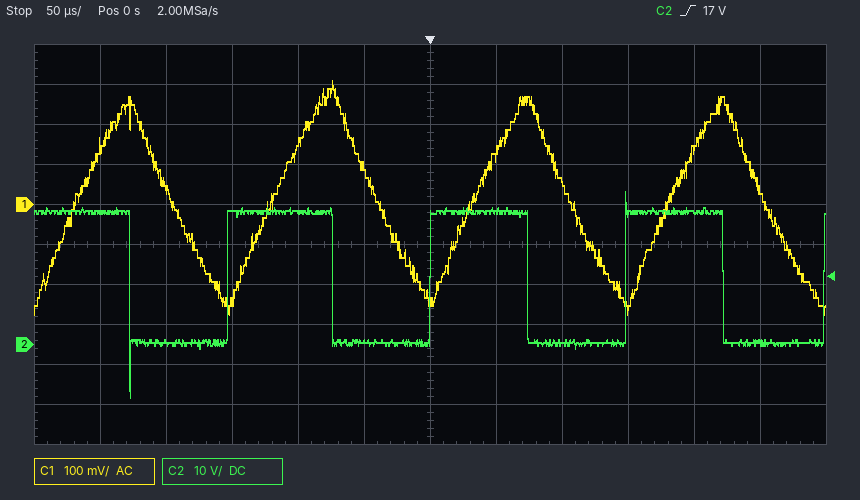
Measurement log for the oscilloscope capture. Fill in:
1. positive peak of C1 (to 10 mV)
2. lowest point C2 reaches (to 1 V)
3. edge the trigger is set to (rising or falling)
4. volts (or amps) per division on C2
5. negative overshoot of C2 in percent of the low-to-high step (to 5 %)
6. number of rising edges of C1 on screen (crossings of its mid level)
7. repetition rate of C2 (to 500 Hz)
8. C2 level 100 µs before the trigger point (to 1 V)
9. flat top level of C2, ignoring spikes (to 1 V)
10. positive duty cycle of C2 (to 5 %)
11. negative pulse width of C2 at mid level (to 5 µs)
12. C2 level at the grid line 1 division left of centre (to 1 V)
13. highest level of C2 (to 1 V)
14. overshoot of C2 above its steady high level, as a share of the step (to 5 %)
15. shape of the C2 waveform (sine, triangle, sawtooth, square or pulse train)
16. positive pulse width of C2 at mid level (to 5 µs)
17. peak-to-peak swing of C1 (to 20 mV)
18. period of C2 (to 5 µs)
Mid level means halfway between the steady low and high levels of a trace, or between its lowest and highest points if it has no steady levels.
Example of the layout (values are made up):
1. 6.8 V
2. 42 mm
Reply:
1. 310 mV
2. -13 V
3. rising
4. 10 V
5. 40 %
6. 4
7. 6.5 kHz
8. 33 V
9. 33 V
10. 50 %
11. 75 µs
12. 1 V
13. 38 V
14. 15 %
15. square
16. 75 µs
17. 580 mV
18. 150 µs
